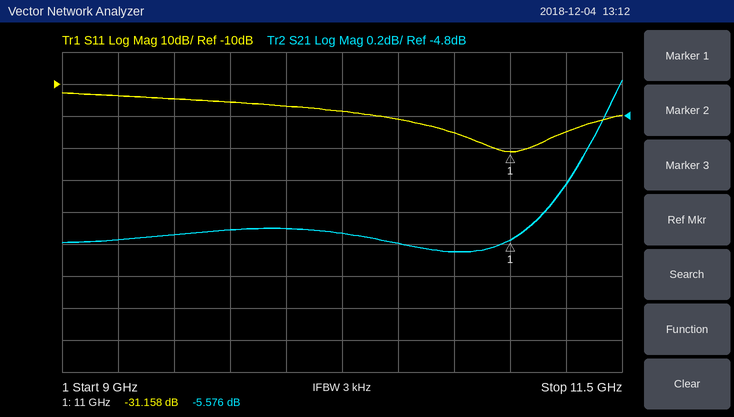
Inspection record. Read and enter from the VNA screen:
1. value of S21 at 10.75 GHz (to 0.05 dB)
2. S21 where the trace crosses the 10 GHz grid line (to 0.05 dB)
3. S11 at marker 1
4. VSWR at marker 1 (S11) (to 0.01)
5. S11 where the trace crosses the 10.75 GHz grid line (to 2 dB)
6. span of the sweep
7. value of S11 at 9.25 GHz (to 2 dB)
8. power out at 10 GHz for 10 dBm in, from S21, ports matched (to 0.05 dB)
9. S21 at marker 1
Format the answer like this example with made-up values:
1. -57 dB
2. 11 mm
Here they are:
1. -5.65 dB
2. -5.50 dB
3. -31.158 dB
4. 1.06
5. -26 dB
6. 2.5 GHz
7. -14 dB
8. 4.50 dBm
9. -5.576 dB
